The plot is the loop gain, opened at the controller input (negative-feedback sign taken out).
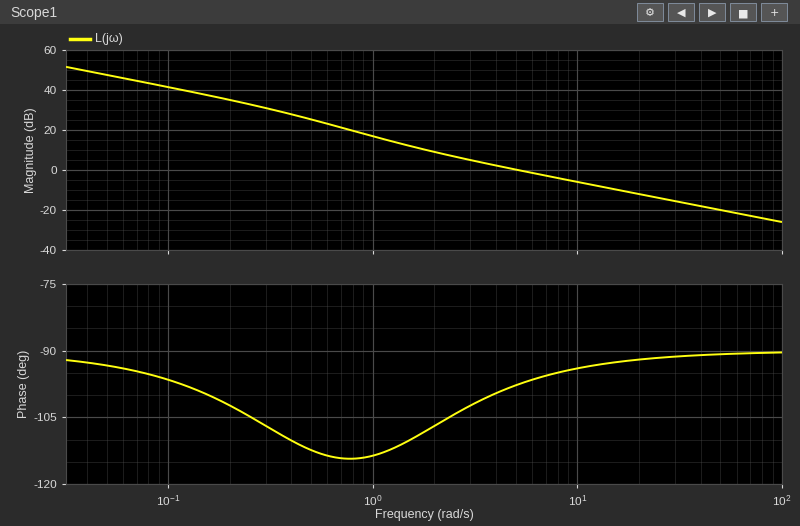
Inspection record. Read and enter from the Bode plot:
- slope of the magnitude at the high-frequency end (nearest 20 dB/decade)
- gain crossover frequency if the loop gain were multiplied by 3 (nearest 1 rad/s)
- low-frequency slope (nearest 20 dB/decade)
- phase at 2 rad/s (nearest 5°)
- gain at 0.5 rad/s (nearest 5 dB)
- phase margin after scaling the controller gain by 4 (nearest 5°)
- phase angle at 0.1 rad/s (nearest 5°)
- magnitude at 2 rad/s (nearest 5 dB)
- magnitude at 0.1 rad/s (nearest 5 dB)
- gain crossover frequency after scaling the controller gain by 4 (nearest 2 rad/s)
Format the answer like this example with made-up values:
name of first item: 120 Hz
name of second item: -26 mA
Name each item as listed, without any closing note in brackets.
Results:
slope of the magnitude at the high-frequency end: -20 dB/decade
gain crossover frequency if the loop gain were multiplied by 3: 15 rad/s
low-frequency slope: -20 dB/decade
phase at 2 rad/s: -105°
gain at 0.5 rad/s: 25 dB
phase margin after scaling the controller gain by 4: 90°
phase angle at 0.1 rad/s: -95°
magnitude at 2 rad/s: 10 dB
magnitude at 0.1 rad/s: 40 dB
gain crossover frequency after scaling the controller gain by 4: 20 rad/s
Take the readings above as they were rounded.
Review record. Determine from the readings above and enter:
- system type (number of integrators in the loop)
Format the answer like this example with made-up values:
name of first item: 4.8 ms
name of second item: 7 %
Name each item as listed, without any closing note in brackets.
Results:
system type: 1
